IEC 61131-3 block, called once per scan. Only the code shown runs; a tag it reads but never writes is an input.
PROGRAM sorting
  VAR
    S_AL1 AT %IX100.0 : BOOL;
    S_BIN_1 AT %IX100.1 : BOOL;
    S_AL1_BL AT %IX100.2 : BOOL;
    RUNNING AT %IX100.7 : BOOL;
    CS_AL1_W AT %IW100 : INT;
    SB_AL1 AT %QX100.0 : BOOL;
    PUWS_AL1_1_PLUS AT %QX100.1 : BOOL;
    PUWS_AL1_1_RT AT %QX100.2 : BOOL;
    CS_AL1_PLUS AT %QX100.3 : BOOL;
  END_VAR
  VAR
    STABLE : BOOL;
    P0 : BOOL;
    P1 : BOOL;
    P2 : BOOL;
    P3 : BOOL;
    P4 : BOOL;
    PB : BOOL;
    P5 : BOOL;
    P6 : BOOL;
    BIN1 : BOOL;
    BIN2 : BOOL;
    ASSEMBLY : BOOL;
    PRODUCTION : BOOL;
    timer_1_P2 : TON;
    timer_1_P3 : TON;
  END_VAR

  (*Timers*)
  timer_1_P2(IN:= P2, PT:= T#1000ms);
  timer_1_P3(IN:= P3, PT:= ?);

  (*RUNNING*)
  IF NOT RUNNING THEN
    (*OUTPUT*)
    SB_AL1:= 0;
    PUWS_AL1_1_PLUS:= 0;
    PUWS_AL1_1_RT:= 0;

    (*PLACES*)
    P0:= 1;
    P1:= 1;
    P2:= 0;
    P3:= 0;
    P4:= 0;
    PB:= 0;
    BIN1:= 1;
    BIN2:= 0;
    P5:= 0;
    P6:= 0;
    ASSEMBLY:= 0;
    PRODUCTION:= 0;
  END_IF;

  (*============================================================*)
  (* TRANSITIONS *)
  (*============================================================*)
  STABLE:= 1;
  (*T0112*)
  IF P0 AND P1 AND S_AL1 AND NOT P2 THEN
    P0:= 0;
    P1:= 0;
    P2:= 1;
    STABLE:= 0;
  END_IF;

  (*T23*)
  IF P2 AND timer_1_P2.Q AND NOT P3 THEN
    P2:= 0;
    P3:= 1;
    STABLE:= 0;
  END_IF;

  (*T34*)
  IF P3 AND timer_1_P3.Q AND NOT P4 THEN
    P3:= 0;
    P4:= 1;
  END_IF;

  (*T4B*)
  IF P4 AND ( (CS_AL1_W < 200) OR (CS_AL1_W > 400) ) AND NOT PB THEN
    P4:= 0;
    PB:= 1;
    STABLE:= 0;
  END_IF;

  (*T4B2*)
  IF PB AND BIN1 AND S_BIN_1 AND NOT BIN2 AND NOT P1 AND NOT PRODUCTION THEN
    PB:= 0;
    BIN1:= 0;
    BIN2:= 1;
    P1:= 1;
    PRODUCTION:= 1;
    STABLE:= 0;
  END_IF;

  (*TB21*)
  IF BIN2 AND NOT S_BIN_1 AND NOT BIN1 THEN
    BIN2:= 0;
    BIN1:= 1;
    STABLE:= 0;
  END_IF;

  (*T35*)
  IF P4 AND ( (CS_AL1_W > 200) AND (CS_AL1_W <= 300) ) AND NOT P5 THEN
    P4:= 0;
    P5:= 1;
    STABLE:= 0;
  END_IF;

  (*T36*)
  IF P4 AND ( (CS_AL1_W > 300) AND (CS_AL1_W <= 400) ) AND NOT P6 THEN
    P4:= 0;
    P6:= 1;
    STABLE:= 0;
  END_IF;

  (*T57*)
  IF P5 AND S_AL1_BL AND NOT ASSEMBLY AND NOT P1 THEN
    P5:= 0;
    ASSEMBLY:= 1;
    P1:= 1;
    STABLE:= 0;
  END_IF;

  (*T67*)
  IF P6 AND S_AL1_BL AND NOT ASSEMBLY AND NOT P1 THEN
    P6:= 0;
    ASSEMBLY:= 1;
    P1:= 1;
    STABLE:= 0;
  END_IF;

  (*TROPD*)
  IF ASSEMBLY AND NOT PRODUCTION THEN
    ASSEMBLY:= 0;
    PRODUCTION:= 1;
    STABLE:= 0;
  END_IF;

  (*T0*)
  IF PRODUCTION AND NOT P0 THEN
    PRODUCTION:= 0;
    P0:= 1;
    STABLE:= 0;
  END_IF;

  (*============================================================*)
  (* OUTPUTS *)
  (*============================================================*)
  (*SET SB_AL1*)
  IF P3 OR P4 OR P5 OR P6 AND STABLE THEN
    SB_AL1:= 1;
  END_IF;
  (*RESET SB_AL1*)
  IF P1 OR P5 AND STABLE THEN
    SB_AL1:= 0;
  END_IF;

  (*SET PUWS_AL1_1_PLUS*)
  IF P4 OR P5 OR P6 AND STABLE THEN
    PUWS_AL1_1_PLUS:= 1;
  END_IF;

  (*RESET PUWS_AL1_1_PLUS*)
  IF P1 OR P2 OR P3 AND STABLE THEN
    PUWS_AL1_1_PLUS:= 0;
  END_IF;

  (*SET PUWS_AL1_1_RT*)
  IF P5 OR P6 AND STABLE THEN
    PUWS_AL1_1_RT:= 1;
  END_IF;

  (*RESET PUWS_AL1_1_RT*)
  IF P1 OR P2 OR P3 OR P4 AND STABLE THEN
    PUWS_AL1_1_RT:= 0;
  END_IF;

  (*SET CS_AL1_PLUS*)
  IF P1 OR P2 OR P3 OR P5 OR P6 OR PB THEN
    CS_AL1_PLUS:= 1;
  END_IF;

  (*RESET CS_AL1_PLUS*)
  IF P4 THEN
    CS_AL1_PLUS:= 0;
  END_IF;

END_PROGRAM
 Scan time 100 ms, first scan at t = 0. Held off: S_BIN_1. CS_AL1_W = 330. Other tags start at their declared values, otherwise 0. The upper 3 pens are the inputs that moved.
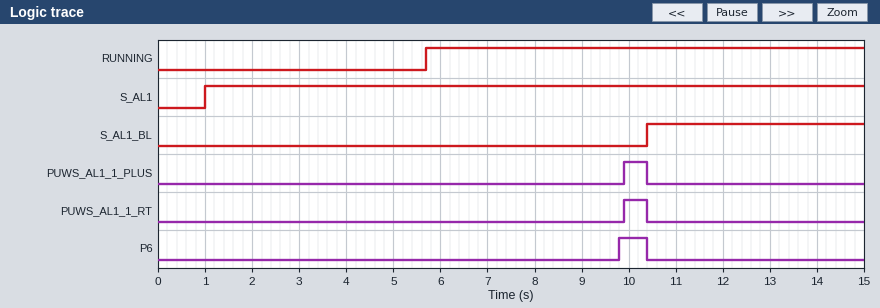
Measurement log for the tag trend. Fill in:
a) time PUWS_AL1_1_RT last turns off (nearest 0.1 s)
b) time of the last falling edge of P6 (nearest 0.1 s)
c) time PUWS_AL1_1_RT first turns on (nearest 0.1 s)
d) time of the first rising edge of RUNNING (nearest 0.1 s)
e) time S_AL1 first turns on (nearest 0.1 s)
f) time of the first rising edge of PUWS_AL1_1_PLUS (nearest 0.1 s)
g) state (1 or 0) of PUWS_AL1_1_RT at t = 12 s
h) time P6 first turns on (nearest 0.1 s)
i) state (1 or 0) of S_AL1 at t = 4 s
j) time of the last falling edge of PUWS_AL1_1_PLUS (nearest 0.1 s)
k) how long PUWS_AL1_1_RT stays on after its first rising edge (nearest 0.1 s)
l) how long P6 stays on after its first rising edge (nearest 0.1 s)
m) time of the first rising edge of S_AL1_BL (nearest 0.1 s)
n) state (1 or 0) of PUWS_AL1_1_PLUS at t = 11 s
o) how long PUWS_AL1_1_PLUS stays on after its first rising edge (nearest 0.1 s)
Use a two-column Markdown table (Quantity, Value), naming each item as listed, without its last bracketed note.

| Quantity | Value |
|---|---|
| time PUWS_AL1_1_RT last turns off | 10.4 s |
| time of the last falling edge of P6 | 10.4 s |
| time PUWS_AL1_1_RT first turns on | 9.9 s |
| time of the first rising edge of RUNNING | 5.7 s |
| time S_AL1 first turns on | 1.0 s |
| time of the first rising edge of PUWS_AL1_1_PLUS | 9.9 s |
| state (1 or 0) of PUWS_AL1_1_RT at t = 12 s | 0 |
| time P6 first turns on | 9.8 s |
| state (1 or 0) of S_AL1 at t = 4 s | 1 |
| time of the last falling edge of PUWS_AL1_1_PLUS | 10.4 s |
| how long PUWS_AL1_1_RT stays on after its first rising edge | 0.5 s |
| how long P6 stays on after its first rising edge | 0.6 s |
| time of the first rising edge of S_AL1_BL | 10.4 s |
| state (1 or 0) of PUWS_AL1_1_PLUS at t = 11 s | 0 |
| how long PUWS_AL1_1_PLUS stays on after its first rising edge | 0.5 s |
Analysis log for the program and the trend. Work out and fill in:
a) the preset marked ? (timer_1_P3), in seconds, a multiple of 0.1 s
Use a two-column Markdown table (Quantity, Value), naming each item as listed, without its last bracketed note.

| Quantity | Value |
|---|---|
| the preset marked ? (timer_1_P3), in seconds, a multiple of 0.1 s | 4.0 s |
